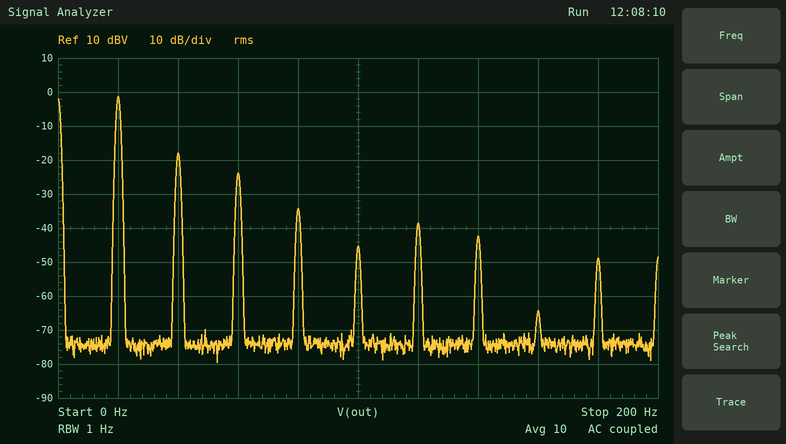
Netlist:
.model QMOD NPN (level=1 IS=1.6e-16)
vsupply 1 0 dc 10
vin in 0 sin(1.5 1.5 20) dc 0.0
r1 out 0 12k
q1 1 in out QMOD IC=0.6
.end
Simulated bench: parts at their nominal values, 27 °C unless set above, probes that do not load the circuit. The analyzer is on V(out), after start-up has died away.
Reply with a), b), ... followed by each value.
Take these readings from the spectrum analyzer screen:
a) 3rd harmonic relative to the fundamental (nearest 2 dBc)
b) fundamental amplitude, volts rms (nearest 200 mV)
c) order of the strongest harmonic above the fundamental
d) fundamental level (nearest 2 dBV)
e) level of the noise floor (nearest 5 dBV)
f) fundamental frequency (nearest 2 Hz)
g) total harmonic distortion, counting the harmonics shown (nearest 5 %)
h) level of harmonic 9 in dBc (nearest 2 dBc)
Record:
a) -22 dBc
b) 800 mV
c) 2
d) -2 dBV
e) -75 dBV
f) 20 Hz
g) 15 %
h) -48 dBc
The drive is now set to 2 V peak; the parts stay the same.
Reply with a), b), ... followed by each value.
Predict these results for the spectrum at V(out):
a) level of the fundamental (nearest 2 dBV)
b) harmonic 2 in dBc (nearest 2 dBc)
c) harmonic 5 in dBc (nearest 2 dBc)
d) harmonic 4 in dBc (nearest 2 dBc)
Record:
a) 0 dBV
b) -14 dBc
c) -32 dBc
d) -56 dBc
